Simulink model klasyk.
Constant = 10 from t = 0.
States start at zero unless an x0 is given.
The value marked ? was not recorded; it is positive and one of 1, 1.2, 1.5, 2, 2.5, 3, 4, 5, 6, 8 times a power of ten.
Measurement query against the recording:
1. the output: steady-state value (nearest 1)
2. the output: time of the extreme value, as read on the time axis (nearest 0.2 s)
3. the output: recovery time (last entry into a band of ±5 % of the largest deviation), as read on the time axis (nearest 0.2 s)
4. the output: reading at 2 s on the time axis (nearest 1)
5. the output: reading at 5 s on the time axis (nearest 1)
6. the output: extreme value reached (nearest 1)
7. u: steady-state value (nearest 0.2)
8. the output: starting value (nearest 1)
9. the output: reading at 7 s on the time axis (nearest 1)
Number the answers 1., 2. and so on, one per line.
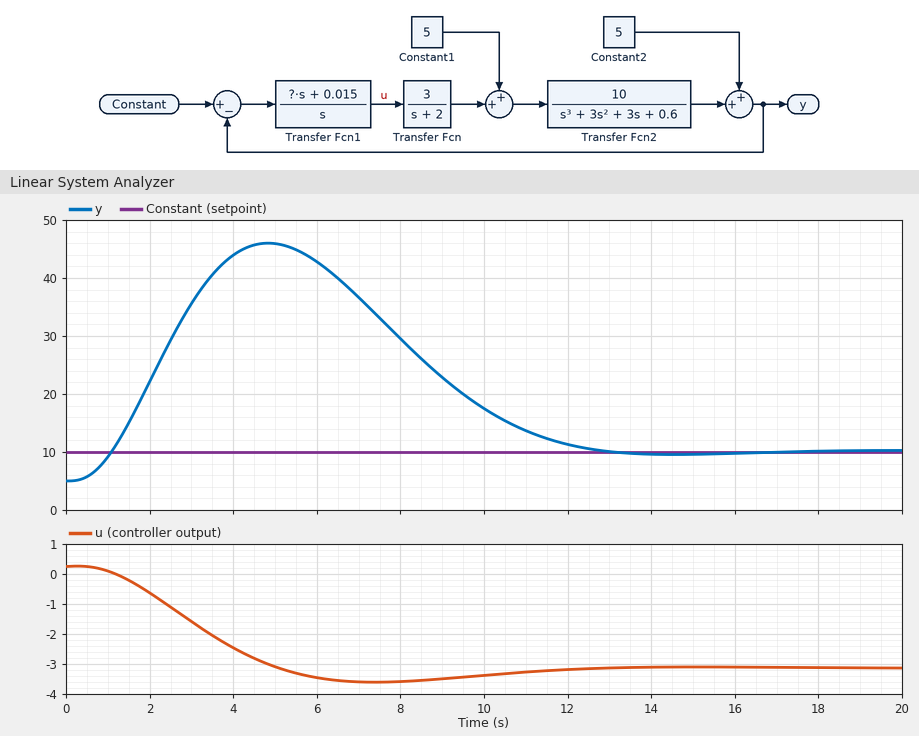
1. 10
2. 4.8 s
3. 11.6 s
4. 22
5. 46
6. 46
7. -3.2
8. 5
9. 37
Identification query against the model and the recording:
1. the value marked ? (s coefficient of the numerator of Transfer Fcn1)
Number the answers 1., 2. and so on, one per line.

1. 0.05
